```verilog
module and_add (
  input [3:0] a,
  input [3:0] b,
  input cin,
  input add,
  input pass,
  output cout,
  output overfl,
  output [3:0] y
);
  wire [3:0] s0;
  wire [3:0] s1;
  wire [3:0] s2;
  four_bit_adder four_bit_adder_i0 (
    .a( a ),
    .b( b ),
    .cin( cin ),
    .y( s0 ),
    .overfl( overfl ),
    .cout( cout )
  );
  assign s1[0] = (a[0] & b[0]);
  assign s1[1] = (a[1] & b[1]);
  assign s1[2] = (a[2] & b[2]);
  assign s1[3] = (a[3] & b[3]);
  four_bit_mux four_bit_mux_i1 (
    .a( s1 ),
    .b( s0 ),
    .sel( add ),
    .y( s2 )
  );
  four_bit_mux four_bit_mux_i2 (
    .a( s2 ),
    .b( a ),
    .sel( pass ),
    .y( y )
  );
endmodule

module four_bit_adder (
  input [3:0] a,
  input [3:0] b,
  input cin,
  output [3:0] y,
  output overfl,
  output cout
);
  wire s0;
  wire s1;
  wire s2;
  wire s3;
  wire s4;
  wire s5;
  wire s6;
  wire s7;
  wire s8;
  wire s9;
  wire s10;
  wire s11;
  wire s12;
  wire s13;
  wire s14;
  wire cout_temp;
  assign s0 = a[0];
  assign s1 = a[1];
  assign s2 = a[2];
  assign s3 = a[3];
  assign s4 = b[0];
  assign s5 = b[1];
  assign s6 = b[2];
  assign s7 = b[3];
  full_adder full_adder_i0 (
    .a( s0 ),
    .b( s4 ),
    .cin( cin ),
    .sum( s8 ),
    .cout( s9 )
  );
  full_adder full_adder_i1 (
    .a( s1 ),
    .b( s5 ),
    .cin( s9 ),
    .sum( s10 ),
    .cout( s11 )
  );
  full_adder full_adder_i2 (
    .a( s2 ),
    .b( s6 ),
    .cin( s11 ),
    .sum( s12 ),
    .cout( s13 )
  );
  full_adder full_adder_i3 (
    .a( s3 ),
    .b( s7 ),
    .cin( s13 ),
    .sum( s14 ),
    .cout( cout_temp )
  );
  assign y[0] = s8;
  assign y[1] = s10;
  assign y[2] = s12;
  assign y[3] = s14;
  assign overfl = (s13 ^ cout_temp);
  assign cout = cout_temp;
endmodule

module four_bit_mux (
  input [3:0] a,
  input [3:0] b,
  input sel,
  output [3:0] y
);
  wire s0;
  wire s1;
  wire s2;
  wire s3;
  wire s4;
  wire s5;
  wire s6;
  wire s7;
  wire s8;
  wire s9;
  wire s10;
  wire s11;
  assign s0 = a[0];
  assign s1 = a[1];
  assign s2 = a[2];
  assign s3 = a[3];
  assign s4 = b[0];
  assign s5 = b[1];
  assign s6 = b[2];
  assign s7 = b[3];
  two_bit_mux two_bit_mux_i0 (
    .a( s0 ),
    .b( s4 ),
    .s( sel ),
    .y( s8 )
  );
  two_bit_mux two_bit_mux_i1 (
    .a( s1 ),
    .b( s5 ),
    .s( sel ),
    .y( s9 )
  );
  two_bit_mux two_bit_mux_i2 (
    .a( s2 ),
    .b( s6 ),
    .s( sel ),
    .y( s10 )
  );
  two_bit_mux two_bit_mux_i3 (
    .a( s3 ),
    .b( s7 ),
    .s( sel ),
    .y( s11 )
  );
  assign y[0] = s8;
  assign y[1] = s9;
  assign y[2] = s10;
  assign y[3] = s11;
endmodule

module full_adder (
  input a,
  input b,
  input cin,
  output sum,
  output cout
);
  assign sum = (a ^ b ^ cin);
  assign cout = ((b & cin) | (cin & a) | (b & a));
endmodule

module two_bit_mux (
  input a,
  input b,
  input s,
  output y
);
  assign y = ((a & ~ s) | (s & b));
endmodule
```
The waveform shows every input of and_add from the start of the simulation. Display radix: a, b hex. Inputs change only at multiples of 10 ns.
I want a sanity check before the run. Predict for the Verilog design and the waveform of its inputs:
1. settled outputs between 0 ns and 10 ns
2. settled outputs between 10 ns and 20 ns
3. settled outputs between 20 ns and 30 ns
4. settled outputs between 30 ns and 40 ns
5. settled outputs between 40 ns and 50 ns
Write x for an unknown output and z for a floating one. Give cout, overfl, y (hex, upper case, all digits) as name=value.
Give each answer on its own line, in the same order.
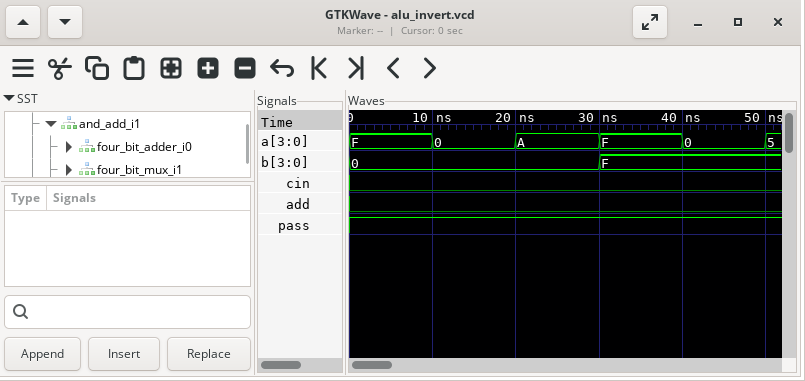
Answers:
cout=0, overfl=0, y=F
cout=0, overfl=0, y=0
cout=0, overfl=0, y=A
cout=1, overfl=0, y=F
cout=0, overfl=0, y=0
